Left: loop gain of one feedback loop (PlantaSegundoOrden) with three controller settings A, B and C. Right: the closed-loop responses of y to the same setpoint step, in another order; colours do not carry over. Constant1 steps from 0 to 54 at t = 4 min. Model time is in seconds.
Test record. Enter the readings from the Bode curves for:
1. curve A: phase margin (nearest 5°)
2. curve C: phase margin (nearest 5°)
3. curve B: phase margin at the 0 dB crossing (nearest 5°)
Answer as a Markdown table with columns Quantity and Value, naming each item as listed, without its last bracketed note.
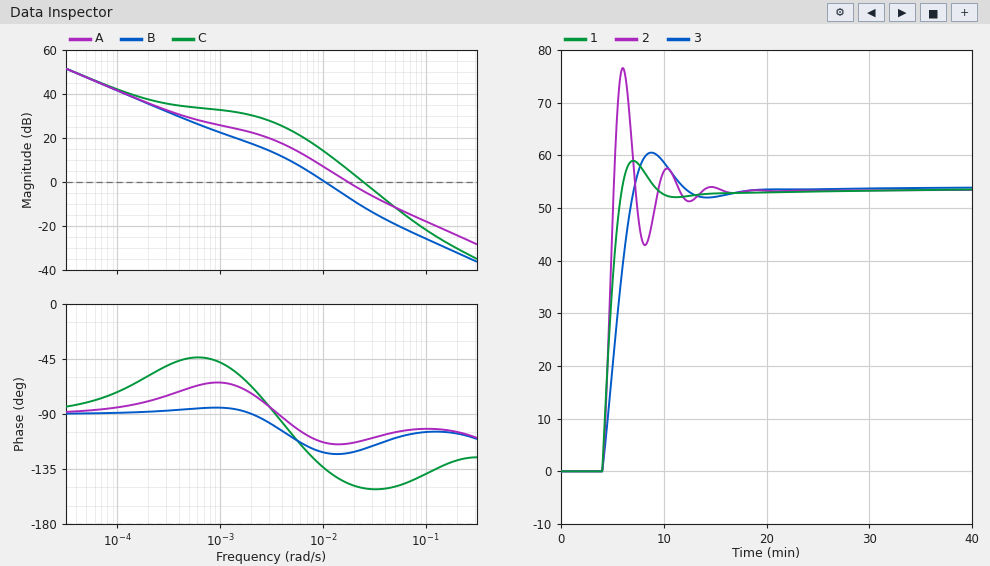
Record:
| Quantity | Value |
|---|---|
| curve A: phase margin | 65° |
| curve C: phase margin | 30° |
| curve B: phase margin at the 0 dB crossing | 60° |
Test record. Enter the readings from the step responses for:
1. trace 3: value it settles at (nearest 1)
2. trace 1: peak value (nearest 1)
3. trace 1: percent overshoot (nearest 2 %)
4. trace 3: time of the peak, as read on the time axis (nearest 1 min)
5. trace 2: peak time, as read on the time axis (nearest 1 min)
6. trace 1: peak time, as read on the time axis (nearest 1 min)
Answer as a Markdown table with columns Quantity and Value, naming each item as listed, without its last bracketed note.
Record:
| Quantity | Value |
|---|---|
| trace 3: value it settles at | 54 |
| trace 1: peak value | 59 |
| trace 1: percent overshoot | 10 % |
| trace 3: time of the peak, as read on the time axis | 9 min |
| trace 2: peak time, as read on the time axis | 6 min |
| trace 1: peak time, as read on the time axis | 7 min |
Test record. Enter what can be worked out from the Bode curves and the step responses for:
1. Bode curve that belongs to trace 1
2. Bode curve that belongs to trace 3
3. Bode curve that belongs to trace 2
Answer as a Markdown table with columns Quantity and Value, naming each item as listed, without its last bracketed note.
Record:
| Quantity | Value |
|---|---|
| Bode curve that belongs to trace 1 | A |
| Bode curve that belongs to trace 3 | B |
| Bode curve that belongs to trace 2 | C |
